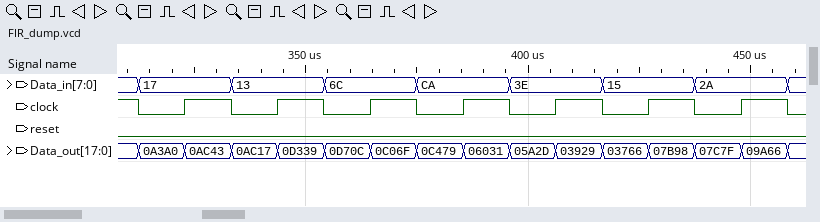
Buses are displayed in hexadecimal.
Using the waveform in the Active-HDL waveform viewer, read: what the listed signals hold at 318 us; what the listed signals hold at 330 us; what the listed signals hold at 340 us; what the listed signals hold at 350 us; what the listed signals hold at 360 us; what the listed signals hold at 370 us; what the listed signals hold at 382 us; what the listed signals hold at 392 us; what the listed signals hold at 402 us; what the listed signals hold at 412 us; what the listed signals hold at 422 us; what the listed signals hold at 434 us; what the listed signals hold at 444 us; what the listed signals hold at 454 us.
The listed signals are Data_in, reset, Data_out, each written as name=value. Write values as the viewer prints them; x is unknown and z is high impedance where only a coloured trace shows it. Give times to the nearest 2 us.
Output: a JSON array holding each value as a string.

["Data_in=17, reset=0, Data_out=0A3A0", "Data_in=17, reset=0, Data_out=0AC43", "Data_in=13, reset=0, Data_out=0AC17", "Data_in=13, reset=0, Data_out=0D339", "Data_in=6C, reset=0, Data_out=0D70C", "Data_in=6C, reset=0, Data_out=0C06F", "Data_in=CA, reset=0, Data_out=0C479", "Data_in=CA, reset=0, Data_out=06031", "Data_in=3E, reset=0, Data_out=05A2D", "Data_in=3E, reset=0, Data_out=03929", "Data_in=15, reset=0, Data_out=03766", "Data_in=15, reset=0, Data_out=07B98", "Data_in=2A, reset=0, Data_out=07C7F", "Data_in=2A, reset=0, Data_out=09A66"]
